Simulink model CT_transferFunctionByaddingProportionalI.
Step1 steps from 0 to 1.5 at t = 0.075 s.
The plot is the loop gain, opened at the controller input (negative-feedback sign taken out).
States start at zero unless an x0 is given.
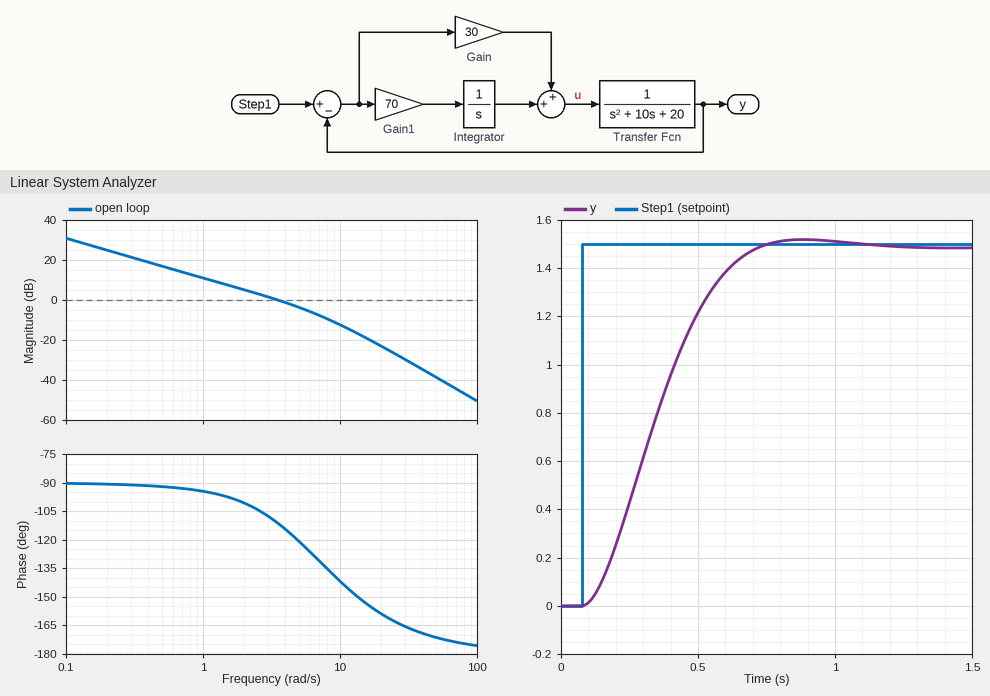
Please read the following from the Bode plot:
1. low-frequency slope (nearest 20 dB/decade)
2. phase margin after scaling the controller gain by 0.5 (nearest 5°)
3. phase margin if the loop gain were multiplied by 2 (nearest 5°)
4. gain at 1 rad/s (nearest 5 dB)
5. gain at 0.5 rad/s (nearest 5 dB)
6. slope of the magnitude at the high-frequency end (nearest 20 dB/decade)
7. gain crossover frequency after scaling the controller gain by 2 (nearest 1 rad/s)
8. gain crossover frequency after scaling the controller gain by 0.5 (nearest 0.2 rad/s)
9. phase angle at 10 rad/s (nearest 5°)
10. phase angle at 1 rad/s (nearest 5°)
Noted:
-20 dB/decade
80°
55°
10 dB
15 dB
-40 dB/decade
6 rad/s
1.8 rad/s
-140°
-95°
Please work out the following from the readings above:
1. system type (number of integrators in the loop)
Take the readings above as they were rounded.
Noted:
1
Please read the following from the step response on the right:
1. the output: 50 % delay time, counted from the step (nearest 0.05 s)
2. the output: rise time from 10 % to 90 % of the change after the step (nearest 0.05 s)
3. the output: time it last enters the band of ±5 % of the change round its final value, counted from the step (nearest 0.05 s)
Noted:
0.25 s
0.40 s
0.55 s
